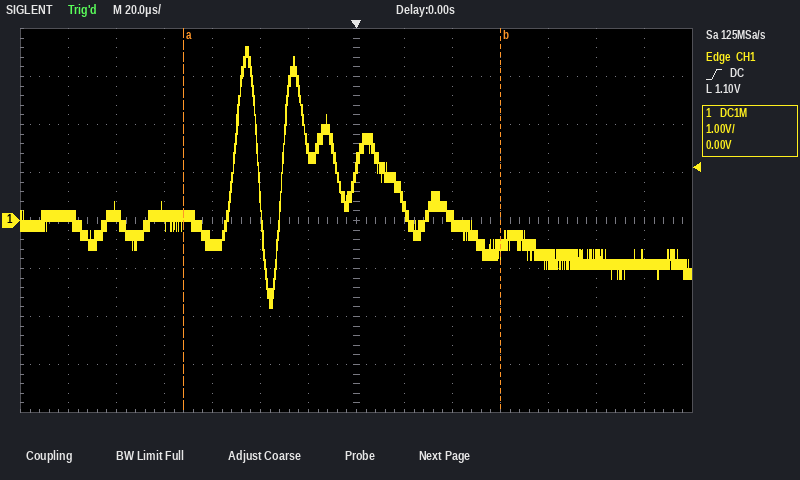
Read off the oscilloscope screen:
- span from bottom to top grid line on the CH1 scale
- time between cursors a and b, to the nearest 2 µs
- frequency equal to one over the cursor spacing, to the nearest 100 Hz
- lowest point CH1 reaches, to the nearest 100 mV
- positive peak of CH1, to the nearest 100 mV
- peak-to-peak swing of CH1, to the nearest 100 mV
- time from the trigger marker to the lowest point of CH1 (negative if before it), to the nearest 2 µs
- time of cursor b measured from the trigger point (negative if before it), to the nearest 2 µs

8 V
132 µs
7.6 kHz
-1.8 V
3.6 V
5.4 V
-36 µs
+60 µs
